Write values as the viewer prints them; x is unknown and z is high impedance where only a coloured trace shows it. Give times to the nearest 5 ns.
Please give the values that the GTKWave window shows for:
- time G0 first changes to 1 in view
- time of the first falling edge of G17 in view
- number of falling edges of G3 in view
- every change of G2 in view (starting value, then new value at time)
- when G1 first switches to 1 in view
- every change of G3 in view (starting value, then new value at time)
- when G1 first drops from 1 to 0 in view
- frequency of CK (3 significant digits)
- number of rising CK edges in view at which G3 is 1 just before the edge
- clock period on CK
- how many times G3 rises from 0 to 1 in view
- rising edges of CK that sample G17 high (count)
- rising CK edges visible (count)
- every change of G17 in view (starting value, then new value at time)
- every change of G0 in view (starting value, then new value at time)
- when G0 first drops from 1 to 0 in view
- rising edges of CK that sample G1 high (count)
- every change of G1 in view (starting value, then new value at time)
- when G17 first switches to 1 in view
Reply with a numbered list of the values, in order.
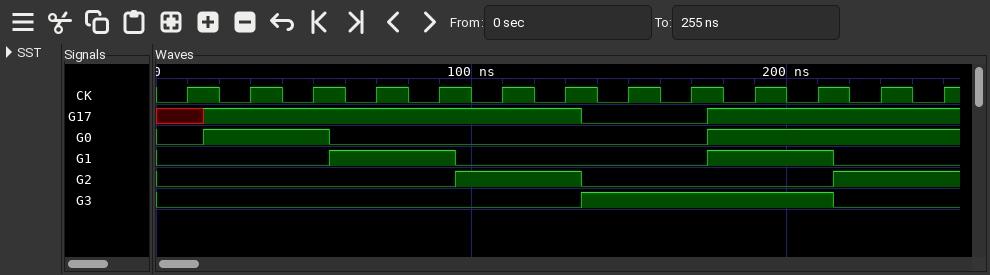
1. 15 ns
2. 135 ns
3. 1
4. 0, 1 at 95 ns, 0 at 135 ns, 1 at 215 ns
5. 55 ns
6. 0, 1 at 135 ns, 0 at 215 ns
7. 95 ns
8. 50.0 MHz
9. 4
10. 20 ns
11. 1
12. 10
13. 13
14. x, 1 at 15 ns, 0 at 135 ns, 1 at 175 ns
15. 0, 1 at 15 ns, 0 at 55 ns, 1 at 175 ns
16. 55 ns
17. 4
18. 0, 1 at 55 ns, 0 at 95 ns, 1 at 175 ns, 0 at 215 ns
19. 15 ns
